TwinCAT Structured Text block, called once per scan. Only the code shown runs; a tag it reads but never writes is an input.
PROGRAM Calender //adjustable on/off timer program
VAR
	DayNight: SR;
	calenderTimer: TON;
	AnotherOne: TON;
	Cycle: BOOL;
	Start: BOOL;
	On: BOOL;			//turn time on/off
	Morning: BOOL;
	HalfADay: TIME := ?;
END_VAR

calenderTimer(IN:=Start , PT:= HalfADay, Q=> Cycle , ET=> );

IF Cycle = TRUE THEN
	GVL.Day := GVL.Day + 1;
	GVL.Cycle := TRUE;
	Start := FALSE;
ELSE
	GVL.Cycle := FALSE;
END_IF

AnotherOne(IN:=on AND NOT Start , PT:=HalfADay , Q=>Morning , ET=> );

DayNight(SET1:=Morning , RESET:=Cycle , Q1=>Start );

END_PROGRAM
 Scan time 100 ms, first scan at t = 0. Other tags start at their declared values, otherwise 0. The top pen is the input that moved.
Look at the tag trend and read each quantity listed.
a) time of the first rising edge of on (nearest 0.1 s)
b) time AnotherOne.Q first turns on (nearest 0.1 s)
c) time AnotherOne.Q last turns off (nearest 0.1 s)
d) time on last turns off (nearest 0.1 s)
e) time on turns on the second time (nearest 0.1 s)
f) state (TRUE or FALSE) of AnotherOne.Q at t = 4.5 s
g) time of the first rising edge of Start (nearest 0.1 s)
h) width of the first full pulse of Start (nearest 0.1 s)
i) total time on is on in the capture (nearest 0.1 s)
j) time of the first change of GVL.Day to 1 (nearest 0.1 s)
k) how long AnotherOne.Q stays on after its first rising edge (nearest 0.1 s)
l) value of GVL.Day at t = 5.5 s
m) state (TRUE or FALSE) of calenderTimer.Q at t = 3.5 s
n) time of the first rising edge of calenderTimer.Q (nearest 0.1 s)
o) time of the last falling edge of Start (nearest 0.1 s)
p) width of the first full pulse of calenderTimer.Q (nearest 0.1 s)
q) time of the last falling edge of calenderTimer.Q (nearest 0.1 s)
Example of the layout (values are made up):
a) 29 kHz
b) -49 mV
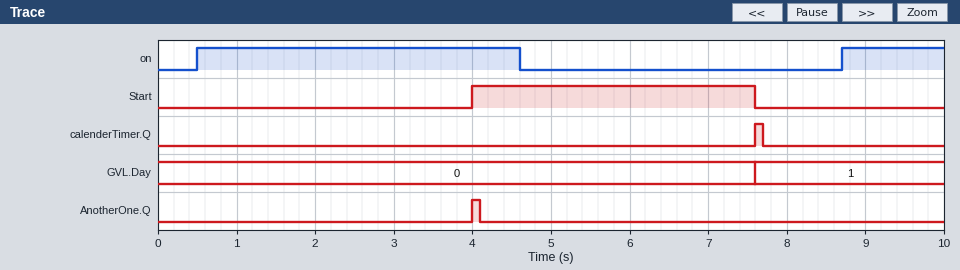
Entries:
a) 0.5 s
b) 4.0 s
c) 4.1 s
d) 4.6 s
e) 8.7 s
f) FALSE
g) 4.0 s
h) 3.6 s
i) 5.4 s
j) 7.6 s
k) 0.1 s
l) 0
m) FALSE
n) 7.6 s
o) 7.6 s
p) 0.1 s
q) 7.7 s
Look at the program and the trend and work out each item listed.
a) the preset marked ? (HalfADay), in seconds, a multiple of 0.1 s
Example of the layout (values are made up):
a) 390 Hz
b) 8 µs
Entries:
a) 3.5 s
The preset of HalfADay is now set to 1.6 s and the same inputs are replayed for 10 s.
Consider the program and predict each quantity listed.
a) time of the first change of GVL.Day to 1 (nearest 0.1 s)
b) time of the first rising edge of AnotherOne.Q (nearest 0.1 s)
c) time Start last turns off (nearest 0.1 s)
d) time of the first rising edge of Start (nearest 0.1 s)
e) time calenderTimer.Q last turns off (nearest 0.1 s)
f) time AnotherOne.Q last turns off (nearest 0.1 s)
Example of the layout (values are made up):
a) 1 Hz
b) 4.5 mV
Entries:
a) 3.8 s
b) 2.1 s
c) 3.8 s
d) 2.1 s
e) 3.9 s
f) 2.2 s
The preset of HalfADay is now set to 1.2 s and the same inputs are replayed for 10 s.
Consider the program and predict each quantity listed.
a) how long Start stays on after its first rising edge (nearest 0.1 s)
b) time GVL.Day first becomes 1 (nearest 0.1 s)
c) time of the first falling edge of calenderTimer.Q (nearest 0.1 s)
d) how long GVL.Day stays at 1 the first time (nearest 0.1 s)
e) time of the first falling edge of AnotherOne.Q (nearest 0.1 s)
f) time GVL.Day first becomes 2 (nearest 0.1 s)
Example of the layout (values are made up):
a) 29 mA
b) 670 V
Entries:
a) 1.3 s
b) 3.0 s
c) 3.1 s
d) 2.5 s
e) 1.8 s
f) 5.5 s
